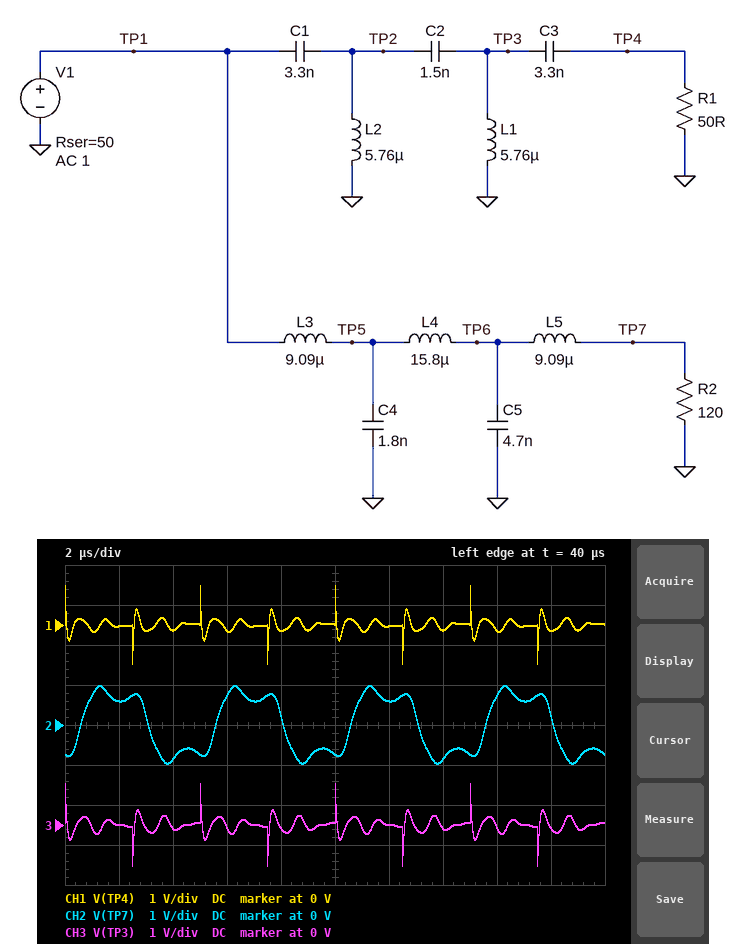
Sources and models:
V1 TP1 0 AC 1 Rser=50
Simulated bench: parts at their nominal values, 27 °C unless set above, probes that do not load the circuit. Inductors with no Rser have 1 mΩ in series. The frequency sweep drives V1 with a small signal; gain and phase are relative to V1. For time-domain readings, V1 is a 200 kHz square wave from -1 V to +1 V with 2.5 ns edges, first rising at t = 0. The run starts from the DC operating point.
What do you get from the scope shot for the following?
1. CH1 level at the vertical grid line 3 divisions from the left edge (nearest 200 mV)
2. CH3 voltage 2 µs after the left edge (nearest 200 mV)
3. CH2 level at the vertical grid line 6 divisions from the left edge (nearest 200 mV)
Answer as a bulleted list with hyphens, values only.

- -200 mV
- 0 V
- 600 mV
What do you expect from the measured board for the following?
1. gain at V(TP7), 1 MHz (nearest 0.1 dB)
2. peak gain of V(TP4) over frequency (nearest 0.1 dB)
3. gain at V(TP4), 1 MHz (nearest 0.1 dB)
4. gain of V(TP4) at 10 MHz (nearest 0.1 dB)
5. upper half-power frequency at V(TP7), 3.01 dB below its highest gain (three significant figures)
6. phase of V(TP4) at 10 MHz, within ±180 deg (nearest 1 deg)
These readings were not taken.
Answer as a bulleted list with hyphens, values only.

- -16.7 dB
- -6.0 dB
- -7.2 dB
- -6.0 dB
- 708 kHz
- 22 deg
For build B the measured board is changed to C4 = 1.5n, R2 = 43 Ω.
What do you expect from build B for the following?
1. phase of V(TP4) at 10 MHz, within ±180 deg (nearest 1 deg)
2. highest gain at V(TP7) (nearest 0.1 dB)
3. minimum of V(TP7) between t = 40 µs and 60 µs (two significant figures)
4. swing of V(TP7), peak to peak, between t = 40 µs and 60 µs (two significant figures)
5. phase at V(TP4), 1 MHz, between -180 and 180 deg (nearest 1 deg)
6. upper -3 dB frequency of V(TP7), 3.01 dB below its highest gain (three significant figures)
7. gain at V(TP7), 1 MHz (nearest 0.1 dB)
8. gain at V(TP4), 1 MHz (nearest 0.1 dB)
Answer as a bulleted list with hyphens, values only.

- 22 deg
- -6.7 dB
- -550 mV
- 1.1 V
- -125 deg
- 728 kHz
- -18.3 dB
- -7.5 dB
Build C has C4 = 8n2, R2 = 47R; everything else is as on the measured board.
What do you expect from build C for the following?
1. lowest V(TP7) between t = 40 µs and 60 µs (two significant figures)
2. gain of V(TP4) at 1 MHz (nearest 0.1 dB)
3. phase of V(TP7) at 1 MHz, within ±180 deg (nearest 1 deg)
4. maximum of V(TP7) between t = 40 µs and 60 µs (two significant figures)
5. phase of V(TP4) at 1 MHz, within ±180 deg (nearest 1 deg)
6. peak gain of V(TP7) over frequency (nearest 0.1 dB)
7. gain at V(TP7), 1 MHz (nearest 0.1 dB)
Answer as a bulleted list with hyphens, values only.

- -570 mV
- -9.7 dB
- 53 deg
- 570 mV
- -107 deg
- -6.3 dB
- -18.1 dB
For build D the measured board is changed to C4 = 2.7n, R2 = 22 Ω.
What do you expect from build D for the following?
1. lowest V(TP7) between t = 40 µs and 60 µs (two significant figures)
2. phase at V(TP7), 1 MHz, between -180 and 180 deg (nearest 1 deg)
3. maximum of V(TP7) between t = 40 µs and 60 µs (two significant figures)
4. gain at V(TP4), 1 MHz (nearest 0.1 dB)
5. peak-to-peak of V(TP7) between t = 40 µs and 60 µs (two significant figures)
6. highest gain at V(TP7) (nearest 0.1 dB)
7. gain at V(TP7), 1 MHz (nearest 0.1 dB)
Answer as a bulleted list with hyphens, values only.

- -340 mV
- 157 deg
- 340 mV
- -8.1 dB
- 680 mV
- -10.3 dB
- -18.0 dB
